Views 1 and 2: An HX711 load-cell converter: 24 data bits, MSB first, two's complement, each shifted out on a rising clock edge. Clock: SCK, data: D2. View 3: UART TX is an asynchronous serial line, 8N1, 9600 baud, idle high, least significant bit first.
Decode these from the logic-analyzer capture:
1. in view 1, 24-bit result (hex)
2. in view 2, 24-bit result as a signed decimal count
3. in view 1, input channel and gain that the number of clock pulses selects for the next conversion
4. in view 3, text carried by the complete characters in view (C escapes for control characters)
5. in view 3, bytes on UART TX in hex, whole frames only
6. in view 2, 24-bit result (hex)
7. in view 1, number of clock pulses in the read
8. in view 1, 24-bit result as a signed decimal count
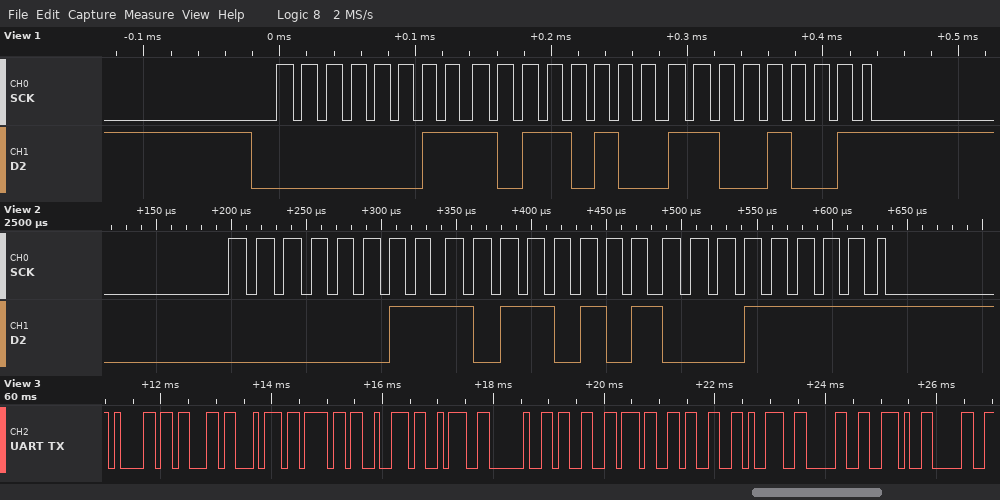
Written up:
0x03B4C9
242975
channel A, gain 128
"actor: 37390.0"
61 63 74 6F 72 3A 20 33 37 33 39 30 2E 30
0x03B51F
25
242889
